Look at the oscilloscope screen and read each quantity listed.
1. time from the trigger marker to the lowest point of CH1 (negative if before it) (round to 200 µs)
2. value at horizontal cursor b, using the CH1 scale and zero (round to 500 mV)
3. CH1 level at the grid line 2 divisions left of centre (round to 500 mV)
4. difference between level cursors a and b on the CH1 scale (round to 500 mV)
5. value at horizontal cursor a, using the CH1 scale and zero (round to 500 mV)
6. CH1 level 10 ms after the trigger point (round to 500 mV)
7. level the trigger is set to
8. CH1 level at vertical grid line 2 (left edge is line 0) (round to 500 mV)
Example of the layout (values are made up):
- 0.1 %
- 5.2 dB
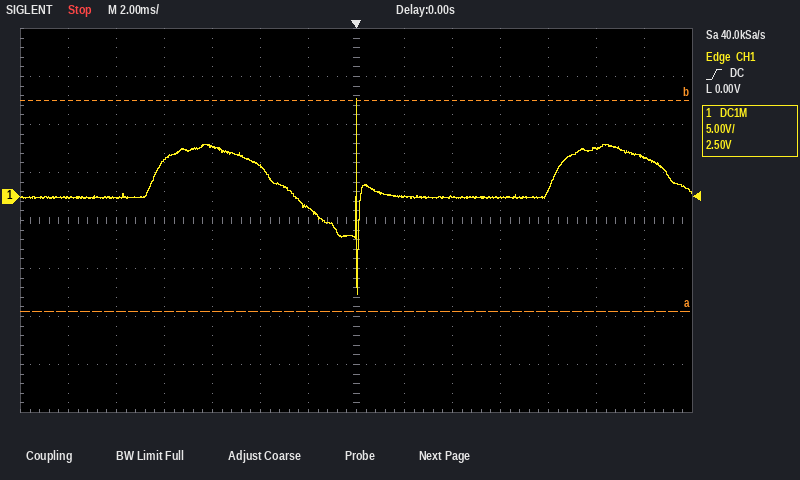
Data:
- 0.0 ms
- 10.0 V
- 3.0 V
- 22.0 V
- -12.0 V
- 5.0 V
- 0.00 V
- 0.0 V
